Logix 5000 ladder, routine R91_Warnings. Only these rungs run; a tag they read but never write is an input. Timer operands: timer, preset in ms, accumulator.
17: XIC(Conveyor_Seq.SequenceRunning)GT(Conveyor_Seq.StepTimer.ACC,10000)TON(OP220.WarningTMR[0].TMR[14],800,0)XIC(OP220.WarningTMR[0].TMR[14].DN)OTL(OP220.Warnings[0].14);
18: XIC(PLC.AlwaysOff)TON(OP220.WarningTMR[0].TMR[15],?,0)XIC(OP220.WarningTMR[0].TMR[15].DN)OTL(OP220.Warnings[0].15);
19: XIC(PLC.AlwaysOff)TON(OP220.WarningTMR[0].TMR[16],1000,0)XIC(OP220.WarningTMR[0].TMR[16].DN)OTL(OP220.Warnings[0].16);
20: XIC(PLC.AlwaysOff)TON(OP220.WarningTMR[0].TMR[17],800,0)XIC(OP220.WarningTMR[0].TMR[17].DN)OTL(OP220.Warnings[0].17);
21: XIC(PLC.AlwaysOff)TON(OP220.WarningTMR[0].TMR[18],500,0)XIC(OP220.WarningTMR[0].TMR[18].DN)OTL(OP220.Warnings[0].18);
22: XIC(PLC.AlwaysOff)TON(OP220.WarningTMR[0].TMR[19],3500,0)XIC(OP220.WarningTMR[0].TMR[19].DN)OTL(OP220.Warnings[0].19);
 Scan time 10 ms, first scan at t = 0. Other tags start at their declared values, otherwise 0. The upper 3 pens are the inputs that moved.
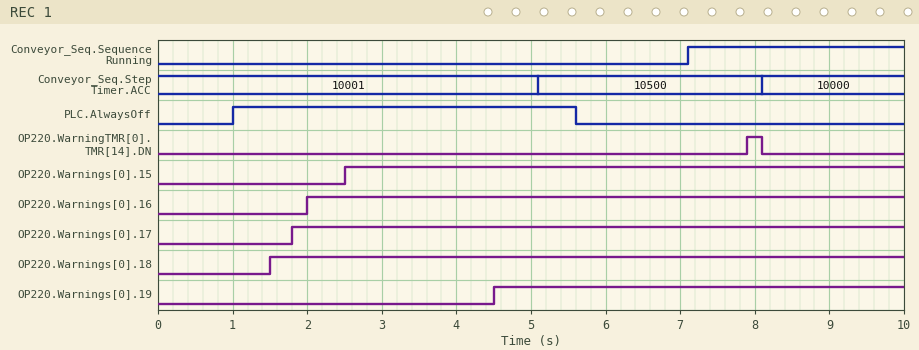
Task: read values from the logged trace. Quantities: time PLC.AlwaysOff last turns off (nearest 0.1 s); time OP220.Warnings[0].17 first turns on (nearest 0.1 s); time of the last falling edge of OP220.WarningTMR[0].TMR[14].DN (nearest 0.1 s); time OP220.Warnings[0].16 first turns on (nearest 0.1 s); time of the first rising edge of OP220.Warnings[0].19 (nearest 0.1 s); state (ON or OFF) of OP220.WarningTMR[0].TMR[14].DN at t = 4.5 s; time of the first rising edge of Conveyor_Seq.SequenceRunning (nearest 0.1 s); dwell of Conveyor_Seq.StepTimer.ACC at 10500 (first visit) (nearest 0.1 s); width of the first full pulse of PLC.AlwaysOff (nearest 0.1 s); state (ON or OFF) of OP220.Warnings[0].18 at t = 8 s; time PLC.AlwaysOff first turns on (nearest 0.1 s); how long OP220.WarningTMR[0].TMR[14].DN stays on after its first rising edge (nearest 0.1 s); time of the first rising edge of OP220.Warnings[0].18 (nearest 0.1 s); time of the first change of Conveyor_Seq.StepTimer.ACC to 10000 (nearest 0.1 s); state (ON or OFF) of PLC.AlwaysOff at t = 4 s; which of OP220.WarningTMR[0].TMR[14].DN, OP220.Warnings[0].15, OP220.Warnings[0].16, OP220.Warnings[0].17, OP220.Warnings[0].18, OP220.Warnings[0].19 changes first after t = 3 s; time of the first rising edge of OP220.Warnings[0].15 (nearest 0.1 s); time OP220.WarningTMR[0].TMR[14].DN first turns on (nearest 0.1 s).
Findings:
5.6 s
1.8 s
8.1 s
2.0 s
4.5 s
OFF
7.1 s
3.0 s
4.6 s
ON
1.0 s
0.2 s
1.5 s
8.1 s
ON
OP220.Warnings[0].19
2.5 s
7.9 s
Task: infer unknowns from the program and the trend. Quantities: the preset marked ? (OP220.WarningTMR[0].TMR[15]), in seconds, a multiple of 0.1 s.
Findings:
1.5 s
